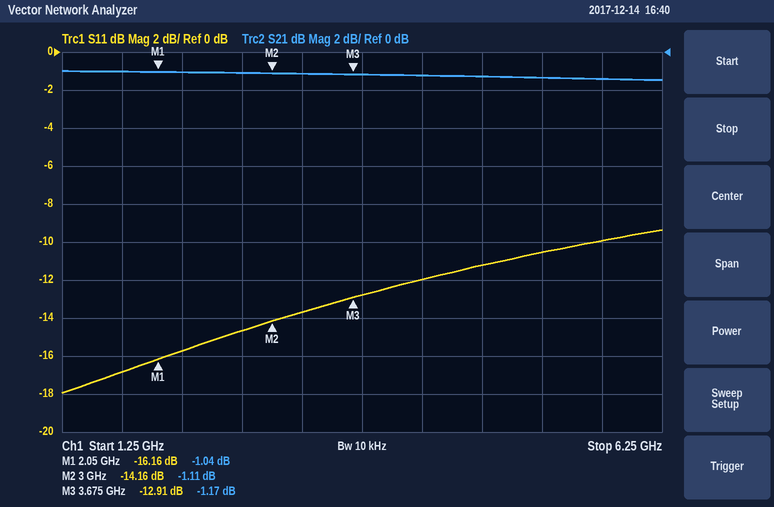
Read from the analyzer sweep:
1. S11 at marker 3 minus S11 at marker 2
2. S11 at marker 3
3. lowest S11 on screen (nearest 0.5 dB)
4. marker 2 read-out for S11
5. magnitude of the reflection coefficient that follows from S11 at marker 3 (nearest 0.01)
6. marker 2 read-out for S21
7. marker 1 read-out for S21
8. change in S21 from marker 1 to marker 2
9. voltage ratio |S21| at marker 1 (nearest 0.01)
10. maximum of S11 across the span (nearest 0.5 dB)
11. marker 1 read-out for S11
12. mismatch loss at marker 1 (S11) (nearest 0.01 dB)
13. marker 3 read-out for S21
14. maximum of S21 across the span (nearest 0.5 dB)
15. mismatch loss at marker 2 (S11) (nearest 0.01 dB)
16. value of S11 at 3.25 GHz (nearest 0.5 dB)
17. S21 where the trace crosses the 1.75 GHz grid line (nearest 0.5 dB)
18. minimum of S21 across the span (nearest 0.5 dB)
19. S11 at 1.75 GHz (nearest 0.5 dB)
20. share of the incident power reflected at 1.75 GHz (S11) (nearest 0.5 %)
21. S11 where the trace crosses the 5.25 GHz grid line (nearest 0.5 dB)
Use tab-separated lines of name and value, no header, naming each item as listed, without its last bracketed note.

S11 at marker 3 minus S11 at marker 2	1.25 dB
S11 at marker 3	-12.91 dB
lowest S11 on screen	-18.0 dB
marker 2 read-out for S11	-14.16 dB
magnitude of the reflection coefficient that follows from S11 at marker 3	0.23
marker 2 read-out for S21	-1.11 dB
marker 1 read-out for S21	-1.04 dB
change in S21 from marker 1 to marker 2	-0.07 dB
voltage ratio |S21| at marker 1	0.89
maximum of S11 across the span	-9.5 dB
marker 1 read-out for S11	-16.16 dB
mismatch loss at marker 1 (S11)	0.11 dB
marker 3 read-out for S21	-1.17 dB
maximum of S21 across the span	-1.0 dB
mismatch loss at marker 2 (S11)	0.17 dB
value of S11 at 3.25 GHz	-13.5 dB
S21 where the trace crosses the 1.75 GHz grid line	-1.0 dB
minimum of S21 across the span	-1.5 dB
S11 at 1.75 GHz	-17.0 dB
share of the incident power reflected at 1.75 GHz (S11)	2.0 %
S11 where the trace crosses the 5.25 GHz grid line	-10.5 dB
